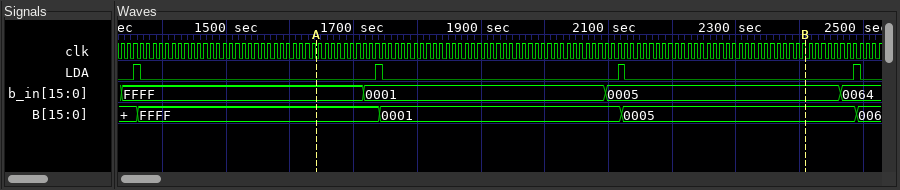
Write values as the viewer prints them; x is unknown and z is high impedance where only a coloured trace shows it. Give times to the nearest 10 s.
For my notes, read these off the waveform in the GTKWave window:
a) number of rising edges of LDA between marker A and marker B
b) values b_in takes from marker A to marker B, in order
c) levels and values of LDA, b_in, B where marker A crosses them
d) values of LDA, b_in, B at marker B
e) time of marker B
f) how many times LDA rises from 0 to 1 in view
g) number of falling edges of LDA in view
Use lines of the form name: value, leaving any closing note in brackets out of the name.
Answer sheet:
number of rising edges of LDA between marker A and marker B: 2
values b_in takes from marker A to marker B, in order: FFFF, 0001, 0005
levels and values of LDA, b_in, B where marker A crosses them: LDA=0, b_in=FFFF, B=FFFF
values of LDA, b_in, B at marker B: LDA=0, b_in=0005, B=0005
time of marker B: 2410 s
how many times LDA rises from 0 to 1 in view: 4
number of falling edges of LDA in view: 4
